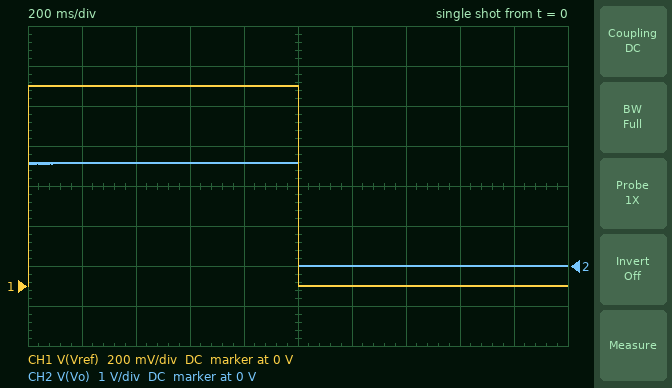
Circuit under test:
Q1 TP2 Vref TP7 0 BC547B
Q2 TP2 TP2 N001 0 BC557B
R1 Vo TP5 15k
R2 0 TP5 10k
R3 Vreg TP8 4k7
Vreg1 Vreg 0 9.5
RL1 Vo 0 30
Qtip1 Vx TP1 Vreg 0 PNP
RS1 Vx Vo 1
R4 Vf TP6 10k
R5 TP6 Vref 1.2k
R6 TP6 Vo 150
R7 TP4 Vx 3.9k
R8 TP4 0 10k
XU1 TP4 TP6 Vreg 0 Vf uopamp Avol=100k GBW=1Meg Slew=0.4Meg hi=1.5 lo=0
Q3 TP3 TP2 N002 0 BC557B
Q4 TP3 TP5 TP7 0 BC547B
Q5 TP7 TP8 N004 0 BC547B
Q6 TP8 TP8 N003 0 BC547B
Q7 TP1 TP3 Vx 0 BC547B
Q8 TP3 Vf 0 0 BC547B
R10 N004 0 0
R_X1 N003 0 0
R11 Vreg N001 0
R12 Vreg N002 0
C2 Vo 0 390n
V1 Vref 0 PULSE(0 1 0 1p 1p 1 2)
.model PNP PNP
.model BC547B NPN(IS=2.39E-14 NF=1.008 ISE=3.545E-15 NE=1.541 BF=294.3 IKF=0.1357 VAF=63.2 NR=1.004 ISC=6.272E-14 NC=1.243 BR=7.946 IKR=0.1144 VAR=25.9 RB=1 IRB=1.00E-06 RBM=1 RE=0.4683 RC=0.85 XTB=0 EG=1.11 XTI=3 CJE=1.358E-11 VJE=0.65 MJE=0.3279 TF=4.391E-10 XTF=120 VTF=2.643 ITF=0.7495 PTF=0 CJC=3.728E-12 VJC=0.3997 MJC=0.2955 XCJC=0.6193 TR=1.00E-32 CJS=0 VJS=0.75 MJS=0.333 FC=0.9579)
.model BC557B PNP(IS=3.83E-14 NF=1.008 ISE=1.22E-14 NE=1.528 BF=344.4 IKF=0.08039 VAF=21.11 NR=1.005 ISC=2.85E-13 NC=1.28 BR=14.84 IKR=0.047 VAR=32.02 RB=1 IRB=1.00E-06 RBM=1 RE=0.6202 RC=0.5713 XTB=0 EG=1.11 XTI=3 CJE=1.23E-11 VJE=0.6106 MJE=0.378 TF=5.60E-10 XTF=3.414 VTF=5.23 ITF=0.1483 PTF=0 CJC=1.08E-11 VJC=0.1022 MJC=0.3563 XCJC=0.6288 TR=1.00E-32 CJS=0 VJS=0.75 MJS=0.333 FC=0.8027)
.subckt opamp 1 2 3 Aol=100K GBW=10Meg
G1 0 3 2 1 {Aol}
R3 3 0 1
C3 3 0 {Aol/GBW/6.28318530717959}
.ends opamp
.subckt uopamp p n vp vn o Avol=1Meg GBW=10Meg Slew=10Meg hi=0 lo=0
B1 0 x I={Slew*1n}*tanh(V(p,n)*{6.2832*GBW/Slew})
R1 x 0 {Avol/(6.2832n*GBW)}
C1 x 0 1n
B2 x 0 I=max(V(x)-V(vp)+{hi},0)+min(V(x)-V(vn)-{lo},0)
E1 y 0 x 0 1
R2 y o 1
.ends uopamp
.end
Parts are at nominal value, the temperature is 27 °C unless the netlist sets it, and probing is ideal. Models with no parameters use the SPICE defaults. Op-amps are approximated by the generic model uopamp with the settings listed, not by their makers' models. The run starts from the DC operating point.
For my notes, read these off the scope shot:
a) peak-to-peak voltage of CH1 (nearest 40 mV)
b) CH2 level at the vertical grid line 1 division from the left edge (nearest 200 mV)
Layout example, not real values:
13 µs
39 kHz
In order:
1.00 V
2.6 V
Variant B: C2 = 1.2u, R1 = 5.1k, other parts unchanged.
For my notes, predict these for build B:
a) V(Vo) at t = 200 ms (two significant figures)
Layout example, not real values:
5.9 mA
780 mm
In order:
1.5 V
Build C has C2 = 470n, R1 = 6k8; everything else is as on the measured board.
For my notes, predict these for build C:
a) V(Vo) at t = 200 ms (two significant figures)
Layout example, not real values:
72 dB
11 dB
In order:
1.7 V
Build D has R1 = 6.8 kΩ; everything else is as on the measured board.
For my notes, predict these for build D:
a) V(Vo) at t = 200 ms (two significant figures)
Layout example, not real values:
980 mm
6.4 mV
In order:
1.7 V
